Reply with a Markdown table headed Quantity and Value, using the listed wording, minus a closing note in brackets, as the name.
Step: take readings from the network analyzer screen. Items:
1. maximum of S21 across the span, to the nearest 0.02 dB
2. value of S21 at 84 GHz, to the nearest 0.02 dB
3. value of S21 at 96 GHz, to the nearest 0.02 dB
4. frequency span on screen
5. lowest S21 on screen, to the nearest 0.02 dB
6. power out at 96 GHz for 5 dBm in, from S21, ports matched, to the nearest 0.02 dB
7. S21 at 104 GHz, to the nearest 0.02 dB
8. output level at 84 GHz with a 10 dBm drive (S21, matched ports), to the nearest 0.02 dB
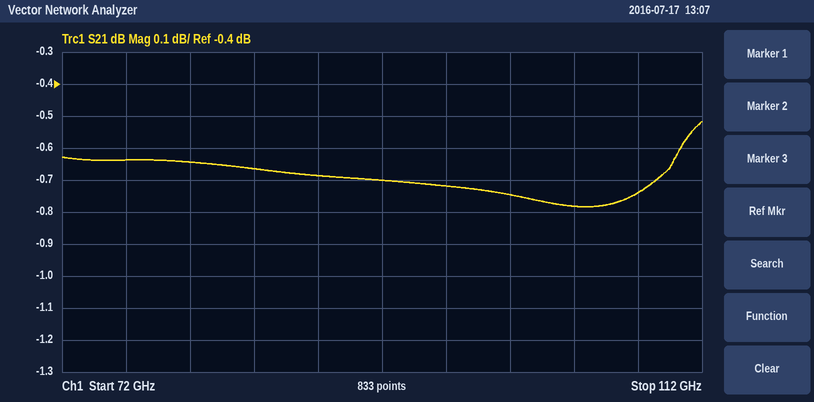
| Quantity | Value |
|---|---|
| maximum of S21 across the span, to the nearest 0.02 dB | -0.52 dB |
| value of S21 at 84 GHz, to the nearest 0.02 dB | -0.66 dB |
| value of S21 at 96 GHz, to the nearest 0.02 dB | -0.72 dB |
| frequency span on screen | 40 GHz |
| lowest S21 on screen, to the nearest 0.02 dB | -0.78 dB |
| power out at 96 GHz for 5 dBm in, from S21, ports matched, to the nearest 0.02 dB | 4.28 dBm |
| S21 at 104 GHz, to the nearest 0.02 dB | -0.78 dB |
| output level at 84 GHz with a 10 dBm drive (S21, matched ports), to the nearest 0.02 dB | 9.34 dBm |
